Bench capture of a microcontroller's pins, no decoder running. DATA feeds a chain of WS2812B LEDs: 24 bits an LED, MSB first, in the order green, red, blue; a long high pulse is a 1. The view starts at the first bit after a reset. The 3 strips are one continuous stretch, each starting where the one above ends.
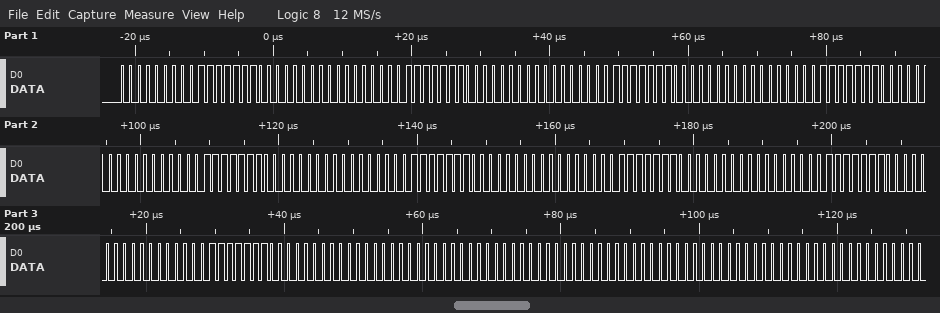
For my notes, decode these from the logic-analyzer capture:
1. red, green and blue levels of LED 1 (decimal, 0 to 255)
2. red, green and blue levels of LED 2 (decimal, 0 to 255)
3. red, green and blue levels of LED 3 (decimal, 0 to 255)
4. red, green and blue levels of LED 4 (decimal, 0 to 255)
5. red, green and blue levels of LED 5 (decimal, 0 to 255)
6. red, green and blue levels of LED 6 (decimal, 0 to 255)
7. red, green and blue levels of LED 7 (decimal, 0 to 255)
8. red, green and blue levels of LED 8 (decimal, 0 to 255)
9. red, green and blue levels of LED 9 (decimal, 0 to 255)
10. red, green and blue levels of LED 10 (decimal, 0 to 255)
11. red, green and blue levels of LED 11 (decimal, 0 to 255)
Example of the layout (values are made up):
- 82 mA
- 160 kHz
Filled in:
- 127, 0, 0
- 127, 0, 0
- 127, 0, 0
- 127, 0, 0
- 127, 0, 0
- 127, 0, 0
- 127, 0, 0
- 127, 0, 0
- 127, 0, 0
- 0, 0, 0
- 0, 0, 0
